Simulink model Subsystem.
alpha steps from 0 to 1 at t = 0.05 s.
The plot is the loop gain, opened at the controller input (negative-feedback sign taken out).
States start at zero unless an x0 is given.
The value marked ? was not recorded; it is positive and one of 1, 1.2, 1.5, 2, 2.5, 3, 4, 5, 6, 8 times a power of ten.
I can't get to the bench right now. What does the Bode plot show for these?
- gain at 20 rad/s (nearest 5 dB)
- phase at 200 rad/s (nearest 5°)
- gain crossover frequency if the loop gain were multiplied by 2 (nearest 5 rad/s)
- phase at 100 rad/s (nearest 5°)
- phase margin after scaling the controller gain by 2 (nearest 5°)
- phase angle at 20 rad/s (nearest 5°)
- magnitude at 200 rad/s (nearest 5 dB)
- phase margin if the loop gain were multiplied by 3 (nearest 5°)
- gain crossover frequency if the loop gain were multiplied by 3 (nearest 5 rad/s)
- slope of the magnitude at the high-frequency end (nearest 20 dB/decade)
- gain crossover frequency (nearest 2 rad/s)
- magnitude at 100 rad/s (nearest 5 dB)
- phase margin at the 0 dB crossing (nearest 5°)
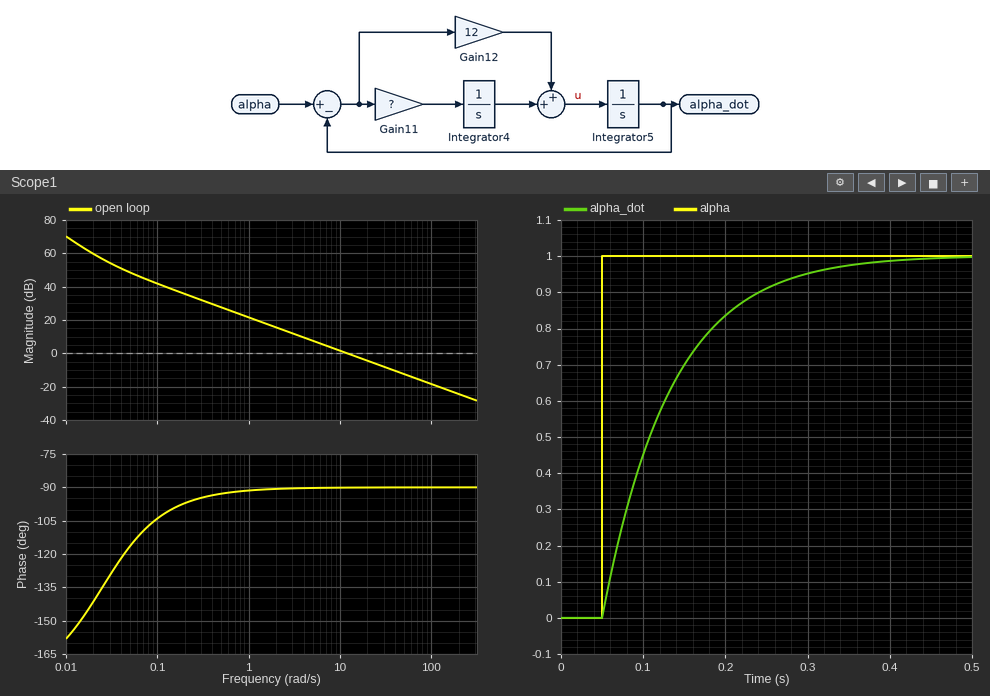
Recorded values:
-5 dB
-90°
25 rad/s
-90°
90°
-90°
-25 dB
90°
35 rad/s
-20 dB/decade
12 rad/s
-20 dB
90°
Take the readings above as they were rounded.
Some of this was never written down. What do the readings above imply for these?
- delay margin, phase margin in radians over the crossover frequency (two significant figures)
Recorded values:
0.13 s
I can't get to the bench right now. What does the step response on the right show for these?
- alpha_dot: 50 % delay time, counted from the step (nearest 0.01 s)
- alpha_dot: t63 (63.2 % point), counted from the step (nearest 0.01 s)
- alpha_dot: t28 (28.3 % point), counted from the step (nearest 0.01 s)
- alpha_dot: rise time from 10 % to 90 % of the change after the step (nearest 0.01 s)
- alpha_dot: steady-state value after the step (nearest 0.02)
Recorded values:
0.06 s
0.08 s
0.03 s
0.18 s
1.00
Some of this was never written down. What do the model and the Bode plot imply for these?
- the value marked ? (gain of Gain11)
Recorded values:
0.3
